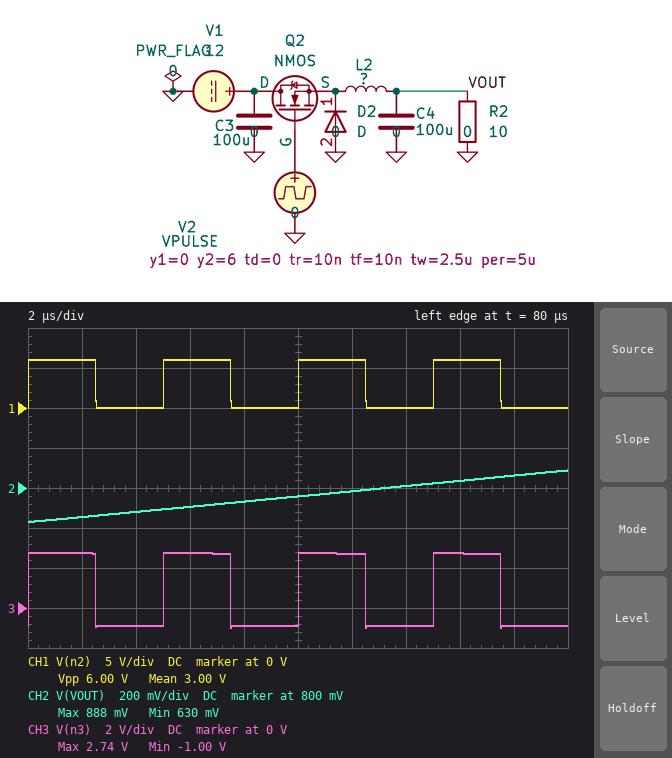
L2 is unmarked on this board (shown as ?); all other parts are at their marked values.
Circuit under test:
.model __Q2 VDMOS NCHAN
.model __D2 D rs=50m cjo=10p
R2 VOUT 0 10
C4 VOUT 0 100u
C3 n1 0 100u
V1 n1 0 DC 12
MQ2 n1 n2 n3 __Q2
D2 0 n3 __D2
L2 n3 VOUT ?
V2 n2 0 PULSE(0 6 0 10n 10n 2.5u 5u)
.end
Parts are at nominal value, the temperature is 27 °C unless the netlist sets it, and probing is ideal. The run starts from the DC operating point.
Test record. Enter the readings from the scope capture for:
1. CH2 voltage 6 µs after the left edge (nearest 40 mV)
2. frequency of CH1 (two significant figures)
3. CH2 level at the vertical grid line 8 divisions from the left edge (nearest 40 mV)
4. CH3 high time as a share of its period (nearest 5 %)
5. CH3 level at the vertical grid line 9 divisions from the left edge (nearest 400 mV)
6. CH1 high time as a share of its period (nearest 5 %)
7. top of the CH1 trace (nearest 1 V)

720 mV
200 kHz
840 mV
50 %
-800 mV
50 %
6 V
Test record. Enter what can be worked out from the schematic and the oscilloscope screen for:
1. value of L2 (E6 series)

47 µH
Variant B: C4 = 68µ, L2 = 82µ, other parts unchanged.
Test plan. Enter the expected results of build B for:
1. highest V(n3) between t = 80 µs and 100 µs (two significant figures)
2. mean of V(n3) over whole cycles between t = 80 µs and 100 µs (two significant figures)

2.8 V
960 mV
